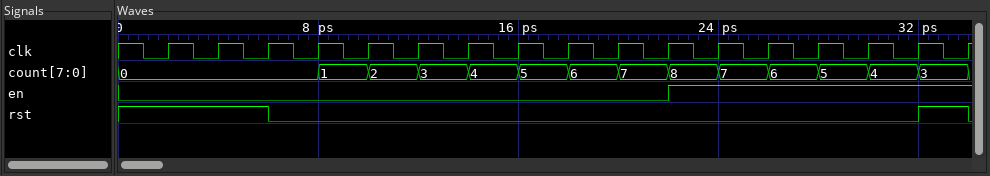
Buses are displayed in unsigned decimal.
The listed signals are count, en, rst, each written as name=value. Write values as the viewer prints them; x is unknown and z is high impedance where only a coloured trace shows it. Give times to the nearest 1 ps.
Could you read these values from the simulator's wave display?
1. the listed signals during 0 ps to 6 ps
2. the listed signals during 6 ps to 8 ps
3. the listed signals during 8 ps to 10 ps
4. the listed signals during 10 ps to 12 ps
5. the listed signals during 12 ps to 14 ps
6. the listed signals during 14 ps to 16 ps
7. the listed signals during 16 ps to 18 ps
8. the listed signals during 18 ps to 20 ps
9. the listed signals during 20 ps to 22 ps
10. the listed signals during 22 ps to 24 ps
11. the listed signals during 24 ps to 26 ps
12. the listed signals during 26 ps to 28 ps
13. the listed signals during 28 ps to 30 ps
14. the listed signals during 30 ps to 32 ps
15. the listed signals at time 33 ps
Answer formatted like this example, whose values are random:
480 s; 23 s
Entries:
count=0, en=0, rst=1; count=0, en=0, rst=0; count=1, en=0, rst=0; count=2, en=0, rst=0; count=3, en=0, rst=0; count=4, en=0, rst=0; count=5, en=0, rst=0; count=6, en=0, rst=0; count=7, en=0, rst=0; count=8, en=1, rst=0; count=7, en=1, rst=0; count=6, en=1, rst=0; count=5, en=1, rst=0; count=4, en=1, rst=0; count=3, en=1, rst=1
